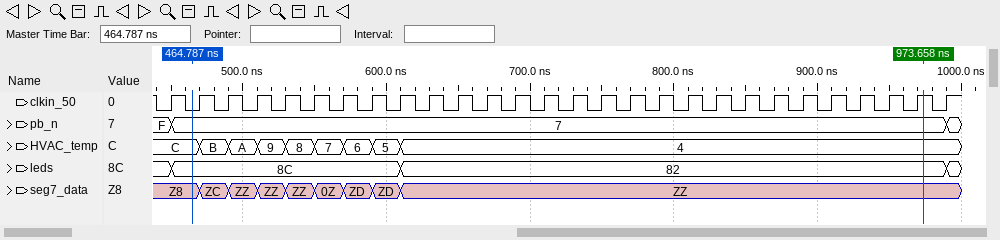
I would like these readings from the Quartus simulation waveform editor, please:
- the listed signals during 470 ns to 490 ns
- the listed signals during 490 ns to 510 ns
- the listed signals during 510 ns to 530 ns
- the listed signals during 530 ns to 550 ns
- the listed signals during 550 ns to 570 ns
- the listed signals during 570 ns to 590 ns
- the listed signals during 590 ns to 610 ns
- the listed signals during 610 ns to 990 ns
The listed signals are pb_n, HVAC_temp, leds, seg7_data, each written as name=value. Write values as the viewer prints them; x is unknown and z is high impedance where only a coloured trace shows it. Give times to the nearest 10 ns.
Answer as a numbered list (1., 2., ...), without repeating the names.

1. pb_n=7, HVAC_temp=B, leds=8C, seg7_data=ZC
2. pb_n=7, HVAC_temp=A, leds=8C, seg7_data=ZZ
3. pb_n=7, HVAC_temp=9, leds=8C, seg7_data=ZZ
4. pb_n=7, HVAC_temp=8, leds=8C, seg7_data=ZZ
5. pb_n=7, HVAC_temp=7, leds=8C, seg7_data=0Z
6. pb_n=7, HVAC_temp=6, leds=8C, seg7_data=ZD
7. pb_n=7, HVAC_temp=5, leds=8C, seg7_data=ZD
8. pb_n=7, HVAC_temp=4, leds=82, seg7_data=ZZ
